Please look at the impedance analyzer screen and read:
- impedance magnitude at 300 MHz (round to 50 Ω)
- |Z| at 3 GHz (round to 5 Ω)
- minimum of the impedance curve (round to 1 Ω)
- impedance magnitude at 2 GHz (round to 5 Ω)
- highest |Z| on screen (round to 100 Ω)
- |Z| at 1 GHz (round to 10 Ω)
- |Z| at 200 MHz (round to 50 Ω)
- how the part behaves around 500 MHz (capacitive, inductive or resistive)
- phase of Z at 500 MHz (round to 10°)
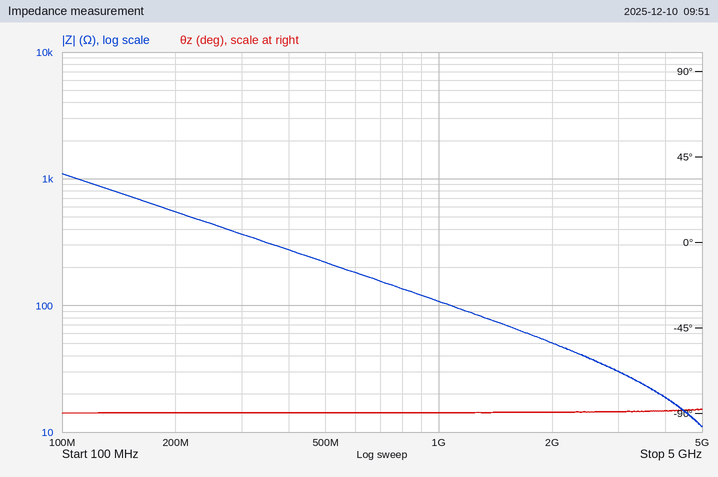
350 Ω
30 Ω
11 Ω
50 Ω
1.1 kΩ
110 Ω
550 Ω
capacitive
-90°
